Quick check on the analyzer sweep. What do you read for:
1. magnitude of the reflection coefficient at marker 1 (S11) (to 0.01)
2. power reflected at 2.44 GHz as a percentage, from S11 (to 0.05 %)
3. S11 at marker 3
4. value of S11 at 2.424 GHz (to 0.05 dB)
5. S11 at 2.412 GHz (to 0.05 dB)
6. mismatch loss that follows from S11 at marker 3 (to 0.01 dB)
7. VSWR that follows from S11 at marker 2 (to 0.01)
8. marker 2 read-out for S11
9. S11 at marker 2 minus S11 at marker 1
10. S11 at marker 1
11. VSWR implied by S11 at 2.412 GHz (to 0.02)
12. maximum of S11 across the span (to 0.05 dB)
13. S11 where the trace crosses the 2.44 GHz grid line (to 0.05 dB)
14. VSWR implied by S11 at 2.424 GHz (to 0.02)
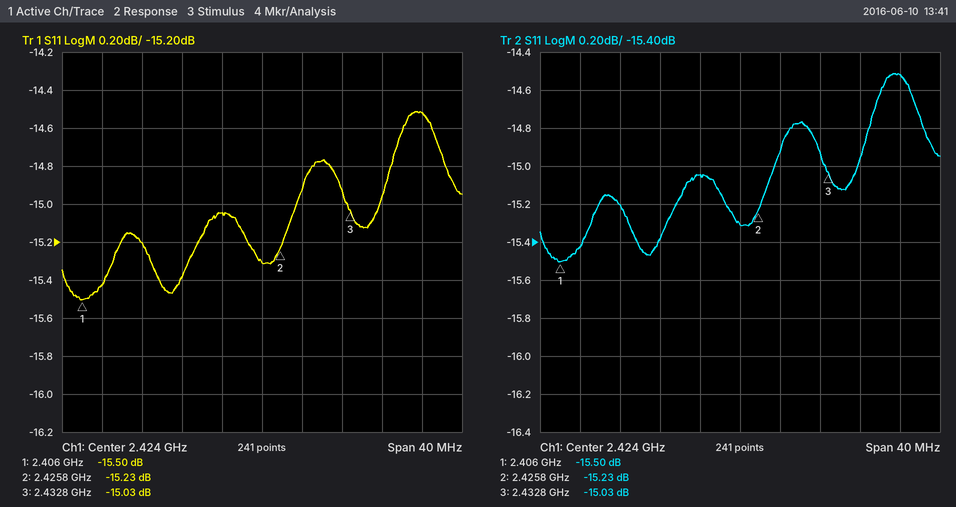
0.17
3.55 %
-15.03 dB
-15.30 dB
-15.20 dB
0.14 dB
1.42
-15.23 dB
0.27 dB
-15.50 dB
1.42
-14.50 dB
-14.50 dB
1.42
